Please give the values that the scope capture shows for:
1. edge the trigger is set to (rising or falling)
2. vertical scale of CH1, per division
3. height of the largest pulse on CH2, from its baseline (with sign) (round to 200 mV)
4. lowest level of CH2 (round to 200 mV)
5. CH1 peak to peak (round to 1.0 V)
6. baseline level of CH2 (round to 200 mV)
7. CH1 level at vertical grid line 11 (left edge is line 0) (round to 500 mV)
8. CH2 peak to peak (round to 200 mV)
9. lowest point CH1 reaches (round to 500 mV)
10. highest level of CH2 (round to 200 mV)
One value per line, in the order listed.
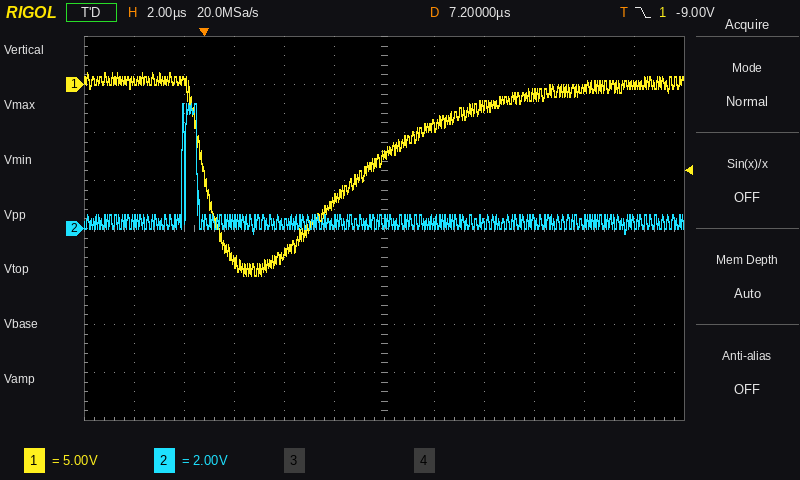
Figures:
falling
5 V
+5.0 V
-200 mV
21.0 V
200 mV
0.0 V
5.4 V
-20.0 V
5.2 V
